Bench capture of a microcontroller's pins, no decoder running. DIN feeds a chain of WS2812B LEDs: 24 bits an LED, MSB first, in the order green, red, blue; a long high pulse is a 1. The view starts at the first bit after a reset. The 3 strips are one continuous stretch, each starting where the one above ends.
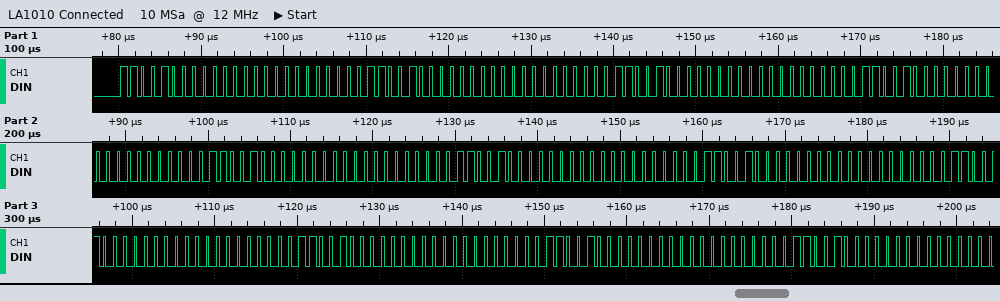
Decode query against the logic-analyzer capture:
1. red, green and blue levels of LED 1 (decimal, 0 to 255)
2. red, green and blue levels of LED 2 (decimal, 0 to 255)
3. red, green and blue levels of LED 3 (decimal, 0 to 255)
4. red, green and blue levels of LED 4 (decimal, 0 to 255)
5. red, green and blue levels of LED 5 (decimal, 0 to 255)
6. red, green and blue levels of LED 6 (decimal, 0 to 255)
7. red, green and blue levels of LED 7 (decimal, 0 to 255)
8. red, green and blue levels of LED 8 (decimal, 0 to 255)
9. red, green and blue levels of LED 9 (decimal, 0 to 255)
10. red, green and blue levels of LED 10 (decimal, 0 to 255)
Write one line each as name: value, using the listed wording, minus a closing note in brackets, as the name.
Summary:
red, green and blue levels of LED 1: 0, 200, 0
red, green and blue levels of LED 2: 0, 200, 0
red, green and blue levels of LED 3: 0, 200, 0
red, green and blue levels of LED 4: 0, 200, 0
red, green and blue levels of LED 5: 0, 200, 0
red, green and blue levels of LED 6: 0, 200, 0
red, green and blue levels of LED 7: 0, 200, 0
red, green and blue levels of LED 8: 0, 200, 0
red, green and blue levels of LED 9: 0, 200, 0
red, green and blue levels of LED 10: 0, 200, 0
